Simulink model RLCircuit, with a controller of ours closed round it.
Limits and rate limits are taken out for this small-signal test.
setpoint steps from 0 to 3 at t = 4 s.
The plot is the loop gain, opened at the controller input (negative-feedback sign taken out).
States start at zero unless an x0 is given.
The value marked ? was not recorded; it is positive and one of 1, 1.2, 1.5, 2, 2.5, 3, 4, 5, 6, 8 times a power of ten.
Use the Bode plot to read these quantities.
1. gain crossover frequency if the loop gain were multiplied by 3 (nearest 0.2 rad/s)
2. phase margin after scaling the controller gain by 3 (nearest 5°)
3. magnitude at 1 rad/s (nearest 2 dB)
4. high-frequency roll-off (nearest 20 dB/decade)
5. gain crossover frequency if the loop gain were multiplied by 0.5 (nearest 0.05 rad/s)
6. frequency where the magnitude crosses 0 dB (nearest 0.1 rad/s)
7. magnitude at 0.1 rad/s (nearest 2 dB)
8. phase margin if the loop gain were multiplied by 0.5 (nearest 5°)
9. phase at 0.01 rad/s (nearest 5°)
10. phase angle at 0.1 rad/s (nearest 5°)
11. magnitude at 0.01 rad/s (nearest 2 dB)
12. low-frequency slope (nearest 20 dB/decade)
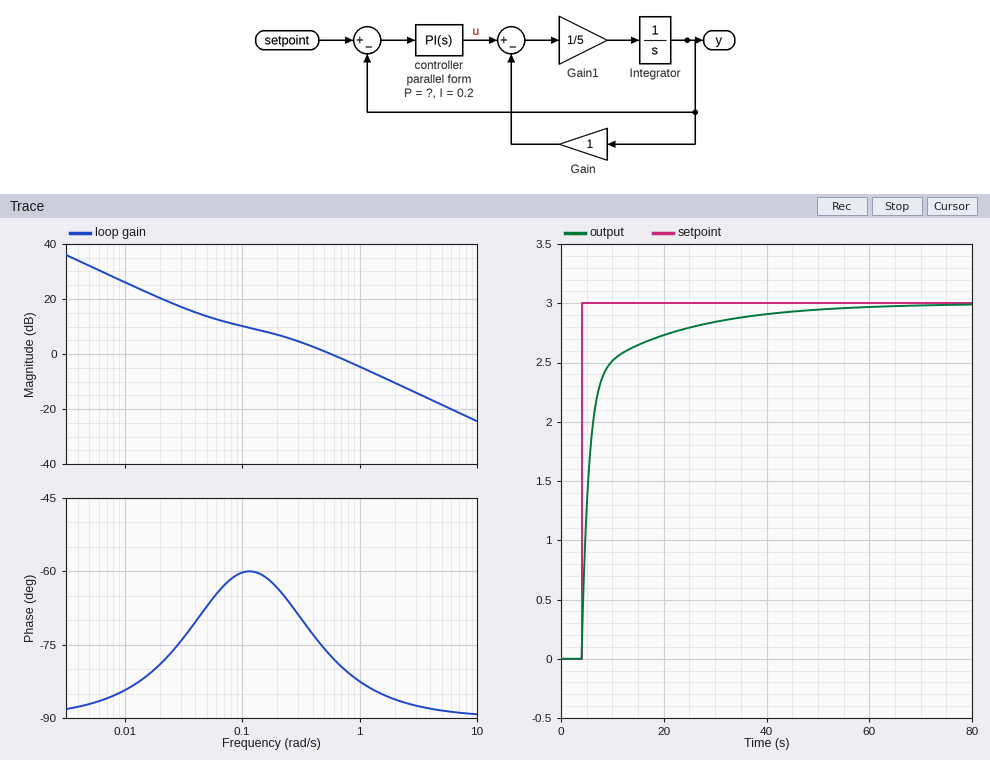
1.8 rad/s
95°
-4 dB
-20 dB/decade
0.25 rad/s
0.6 rad/s
10 dB
115°
-85°
-60°
26 dB
-20 dB/decade
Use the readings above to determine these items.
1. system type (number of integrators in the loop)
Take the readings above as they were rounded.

1
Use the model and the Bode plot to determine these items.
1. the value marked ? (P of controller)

3
